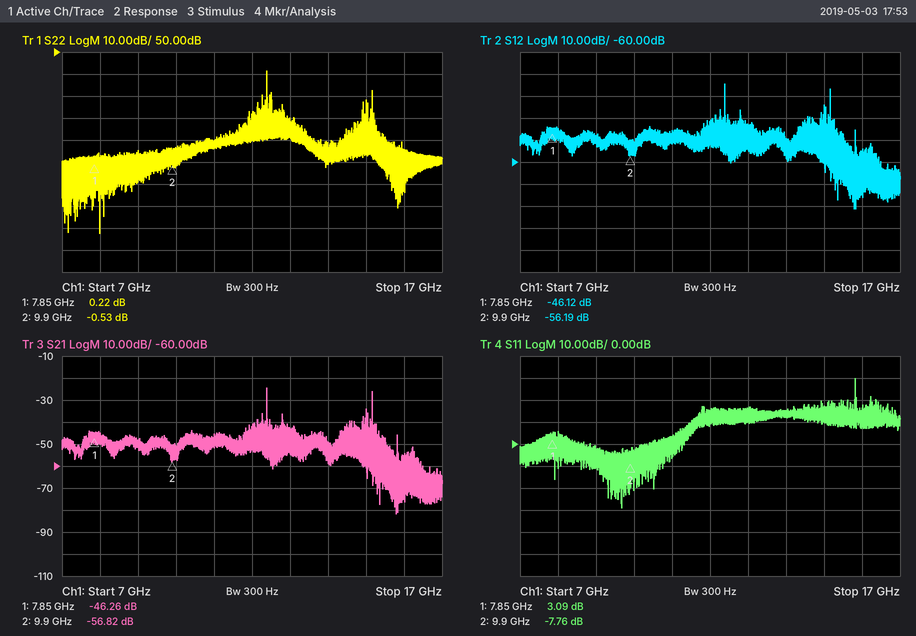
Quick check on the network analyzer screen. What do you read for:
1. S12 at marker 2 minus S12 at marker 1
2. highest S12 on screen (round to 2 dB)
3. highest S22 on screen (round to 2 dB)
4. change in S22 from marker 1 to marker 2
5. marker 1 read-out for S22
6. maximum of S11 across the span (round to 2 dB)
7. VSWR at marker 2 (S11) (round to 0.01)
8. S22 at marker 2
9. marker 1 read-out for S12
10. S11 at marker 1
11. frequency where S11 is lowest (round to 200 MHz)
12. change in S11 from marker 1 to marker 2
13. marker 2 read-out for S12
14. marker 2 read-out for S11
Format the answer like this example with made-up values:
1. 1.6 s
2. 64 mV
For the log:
1. -10.07 dB
2. -24 dB
3. 42 dB
4. -0.75 dB
5. 0.22 dB
6. 30 dB
7. 2.39
8. -0.53 dB
9. -46.12 dB
10. 3.09 dB
11. 9.6 GHz
12. -10.85 dB
13. -56.19 dB
14. -7.76 dB
